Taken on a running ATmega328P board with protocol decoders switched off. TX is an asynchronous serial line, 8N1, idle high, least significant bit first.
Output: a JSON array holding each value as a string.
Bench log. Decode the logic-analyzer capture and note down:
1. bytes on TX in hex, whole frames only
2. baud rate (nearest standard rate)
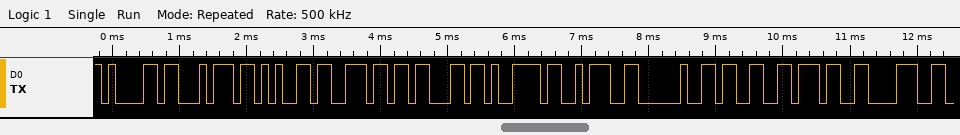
["0x61 0x74 0x65 0x6E 0x63 0x79 0x3A 0x20 0x33 0x37 0x38", "9600 baud"]
